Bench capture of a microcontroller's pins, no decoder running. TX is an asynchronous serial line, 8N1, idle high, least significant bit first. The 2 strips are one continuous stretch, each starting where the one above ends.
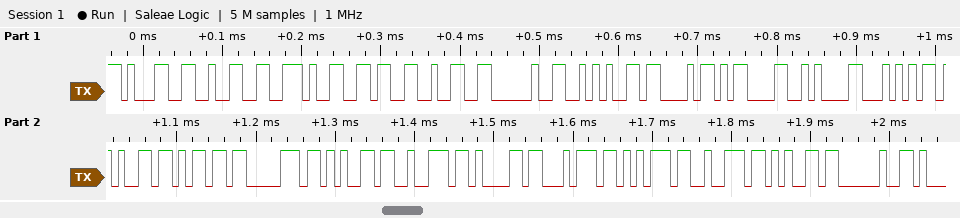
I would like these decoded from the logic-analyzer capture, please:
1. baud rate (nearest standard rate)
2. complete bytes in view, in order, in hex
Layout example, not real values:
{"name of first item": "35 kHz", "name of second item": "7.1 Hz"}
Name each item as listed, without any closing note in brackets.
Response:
{"baud rate": "115200 baud", "complete bytes in view, in order, in hex": "31 32 2E 36 32 20 2A 43 0D 0A 54 65 6D 70 65 72 61 74 75 72 65 20"}
